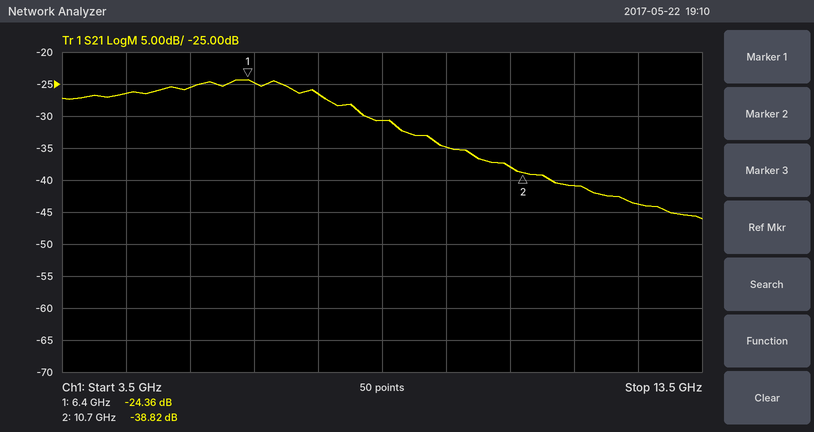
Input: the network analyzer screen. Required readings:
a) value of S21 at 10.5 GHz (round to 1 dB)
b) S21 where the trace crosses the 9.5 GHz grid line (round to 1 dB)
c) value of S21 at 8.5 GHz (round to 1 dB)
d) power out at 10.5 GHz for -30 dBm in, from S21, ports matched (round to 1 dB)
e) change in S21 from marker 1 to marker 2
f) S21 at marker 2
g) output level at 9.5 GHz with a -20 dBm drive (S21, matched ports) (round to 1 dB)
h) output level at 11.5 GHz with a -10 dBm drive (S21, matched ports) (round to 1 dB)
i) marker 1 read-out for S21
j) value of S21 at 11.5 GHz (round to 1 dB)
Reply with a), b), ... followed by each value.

a) -38 dB
b) -35 dB
c) -31 dB
d) -68 dBm
e) -14.46 dB
f) -38.82 dB
g) -55 dBm
h) -51 dBm
i) -24.36 dB
j) -41 dB
